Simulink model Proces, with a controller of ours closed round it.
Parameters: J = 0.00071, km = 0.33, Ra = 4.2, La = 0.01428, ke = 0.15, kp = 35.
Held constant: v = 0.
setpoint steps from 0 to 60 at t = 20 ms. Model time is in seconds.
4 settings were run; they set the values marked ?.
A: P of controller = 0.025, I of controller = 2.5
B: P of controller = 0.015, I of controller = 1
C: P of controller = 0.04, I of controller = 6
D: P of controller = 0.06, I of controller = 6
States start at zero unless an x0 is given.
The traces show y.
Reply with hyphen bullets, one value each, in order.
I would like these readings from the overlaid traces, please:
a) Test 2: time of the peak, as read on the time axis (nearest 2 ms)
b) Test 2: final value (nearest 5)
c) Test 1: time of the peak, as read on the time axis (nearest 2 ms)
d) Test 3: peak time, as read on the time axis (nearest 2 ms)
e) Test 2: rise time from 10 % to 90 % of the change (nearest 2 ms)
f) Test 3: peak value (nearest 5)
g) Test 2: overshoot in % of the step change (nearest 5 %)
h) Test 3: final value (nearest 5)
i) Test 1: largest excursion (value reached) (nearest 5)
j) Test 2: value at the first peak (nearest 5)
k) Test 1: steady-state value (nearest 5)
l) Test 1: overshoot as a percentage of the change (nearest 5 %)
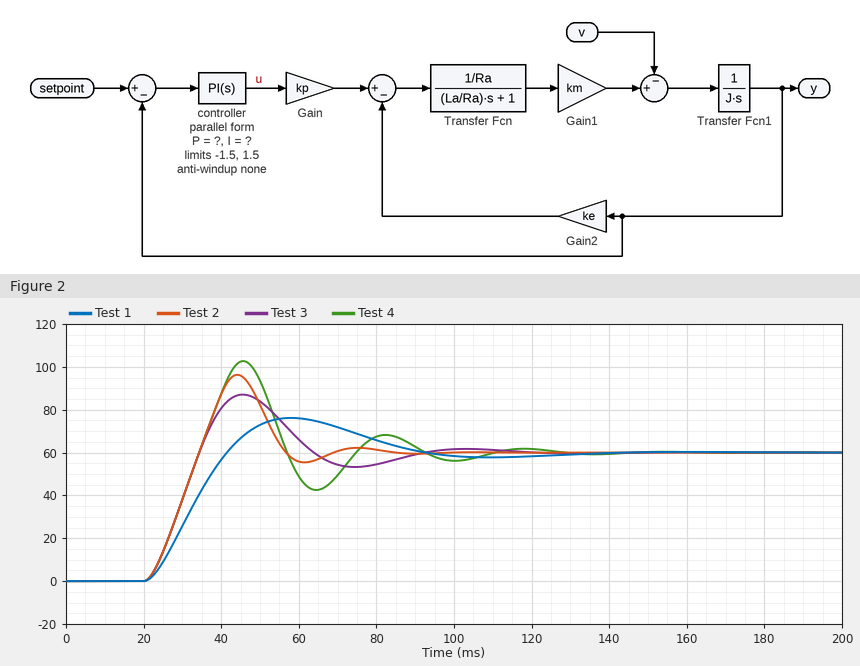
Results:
- 44 ms
- 60
- 58 ms
- 46 ms
- 10 ms
- 85
- 60 %
- 60
- 75
- 95
- 60
- 25 %
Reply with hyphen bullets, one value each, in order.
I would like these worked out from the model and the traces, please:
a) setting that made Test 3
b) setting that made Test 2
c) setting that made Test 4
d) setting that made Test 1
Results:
- A
- D
- C
- B
